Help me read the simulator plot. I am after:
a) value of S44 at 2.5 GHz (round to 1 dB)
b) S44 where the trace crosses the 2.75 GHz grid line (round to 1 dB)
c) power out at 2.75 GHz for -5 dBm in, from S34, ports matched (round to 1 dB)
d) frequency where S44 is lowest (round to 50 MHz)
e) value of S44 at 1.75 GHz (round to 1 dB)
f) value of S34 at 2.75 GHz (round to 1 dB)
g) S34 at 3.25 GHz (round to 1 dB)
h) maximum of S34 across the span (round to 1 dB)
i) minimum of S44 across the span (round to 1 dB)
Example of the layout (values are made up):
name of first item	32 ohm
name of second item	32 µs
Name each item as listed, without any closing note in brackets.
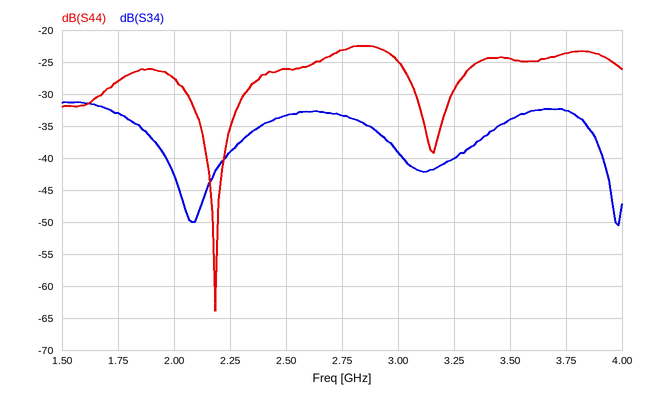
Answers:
value of S44 at 2.5 GHz	-26 dB
S44 where the trace crosses the 2.75 GHz grid line	-23 dB
power out at 2.75 GHz for -5 dBm in, from S34, ports matched	-38 dBm
frequency where S44 is lowest	2.20 GHz
value of S44 at 1.75 GHz	-28 dB
value of S34 at 2.75 GHz	-33 dB
S34 at 3.25 GHz	-40 dB
maximum of S34 across the span	-31 dB
minimum of S44 across the span	-64 dB
